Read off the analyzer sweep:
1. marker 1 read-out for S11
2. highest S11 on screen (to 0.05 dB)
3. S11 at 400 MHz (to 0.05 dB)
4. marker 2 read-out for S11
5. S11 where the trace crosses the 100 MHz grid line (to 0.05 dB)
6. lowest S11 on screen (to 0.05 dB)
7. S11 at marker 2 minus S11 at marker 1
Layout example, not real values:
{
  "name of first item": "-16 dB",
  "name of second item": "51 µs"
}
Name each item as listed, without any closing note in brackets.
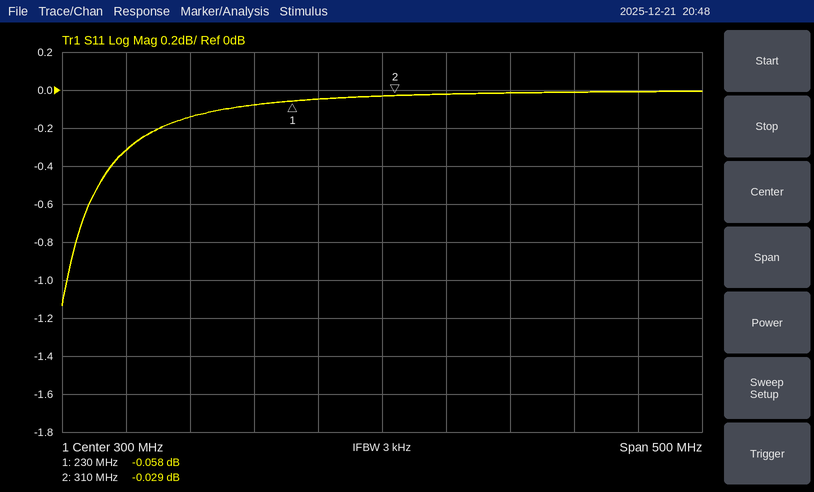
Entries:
{
  "marker 1 read-out for S11": "-0.058 dB",
  "highest S11 on screen": "0.00 dB",
  "S11 at 400 MHz": "0.00 dB",
  "marker 2 read-out for S11": "-0.029 dB",
  "S11 where the trace crosses the 100 MHz grid line": "-0.30 dB",
  "lowest S11 on screen": "-1.15 dB",
  "S11 at marker 2 minus S11 at marker 1": "0.029 dB"
}
